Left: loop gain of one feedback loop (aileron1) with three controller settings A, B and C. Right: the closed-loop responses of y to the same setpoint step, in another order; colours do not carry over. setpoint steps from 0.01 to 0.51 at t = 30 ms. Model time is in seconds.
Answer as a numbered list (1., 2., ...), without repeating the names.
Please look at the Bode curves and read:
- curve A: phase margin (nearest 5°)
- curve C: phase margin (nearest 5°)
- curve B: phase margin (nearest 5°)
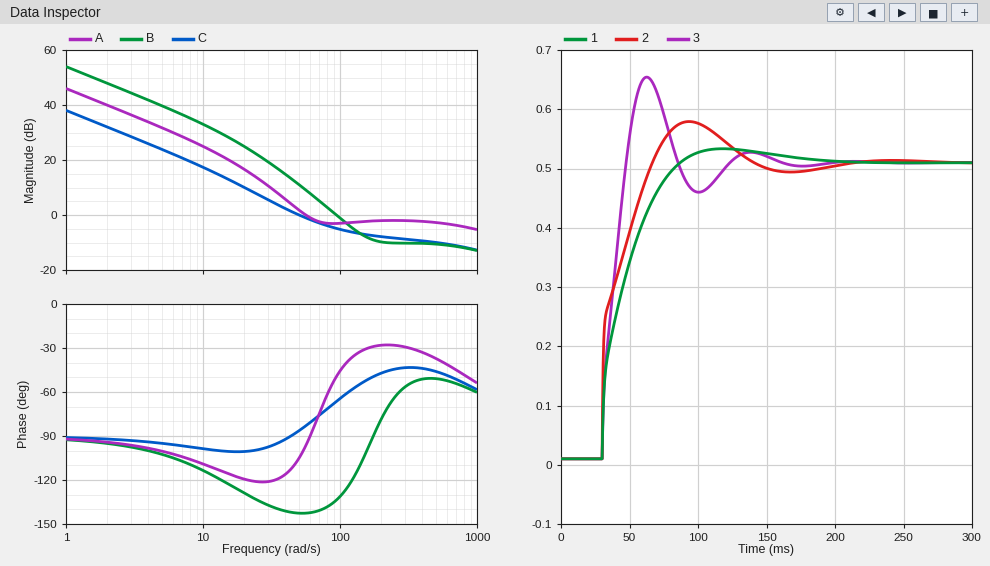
1. 85°
2. 95°
3. 45°
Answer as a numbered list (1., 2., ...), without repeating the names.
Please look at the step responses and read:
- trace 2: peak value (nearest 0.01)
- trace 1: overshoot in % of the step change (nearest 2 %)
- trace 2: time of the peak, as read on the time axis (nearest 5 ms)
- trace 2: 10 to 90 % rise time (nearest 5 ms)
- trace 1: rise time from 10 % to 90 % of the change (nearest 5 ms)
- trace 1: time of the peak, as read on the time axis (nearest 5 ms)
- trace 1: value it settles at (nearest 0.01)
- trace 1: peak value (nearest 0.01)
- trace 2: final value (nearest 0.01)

1. 0.58
2. 4 %
3. 95 ms
4. 30 ms
5. 40 ms
6. 120 ms
7. 0.51
8. 0.53
9. 0.51
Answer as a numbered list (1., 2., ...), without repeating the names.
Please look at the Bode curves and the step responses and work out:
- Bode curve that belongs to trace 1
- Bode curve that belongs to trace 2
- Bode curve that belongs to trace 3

1. C
2. A
3. B
